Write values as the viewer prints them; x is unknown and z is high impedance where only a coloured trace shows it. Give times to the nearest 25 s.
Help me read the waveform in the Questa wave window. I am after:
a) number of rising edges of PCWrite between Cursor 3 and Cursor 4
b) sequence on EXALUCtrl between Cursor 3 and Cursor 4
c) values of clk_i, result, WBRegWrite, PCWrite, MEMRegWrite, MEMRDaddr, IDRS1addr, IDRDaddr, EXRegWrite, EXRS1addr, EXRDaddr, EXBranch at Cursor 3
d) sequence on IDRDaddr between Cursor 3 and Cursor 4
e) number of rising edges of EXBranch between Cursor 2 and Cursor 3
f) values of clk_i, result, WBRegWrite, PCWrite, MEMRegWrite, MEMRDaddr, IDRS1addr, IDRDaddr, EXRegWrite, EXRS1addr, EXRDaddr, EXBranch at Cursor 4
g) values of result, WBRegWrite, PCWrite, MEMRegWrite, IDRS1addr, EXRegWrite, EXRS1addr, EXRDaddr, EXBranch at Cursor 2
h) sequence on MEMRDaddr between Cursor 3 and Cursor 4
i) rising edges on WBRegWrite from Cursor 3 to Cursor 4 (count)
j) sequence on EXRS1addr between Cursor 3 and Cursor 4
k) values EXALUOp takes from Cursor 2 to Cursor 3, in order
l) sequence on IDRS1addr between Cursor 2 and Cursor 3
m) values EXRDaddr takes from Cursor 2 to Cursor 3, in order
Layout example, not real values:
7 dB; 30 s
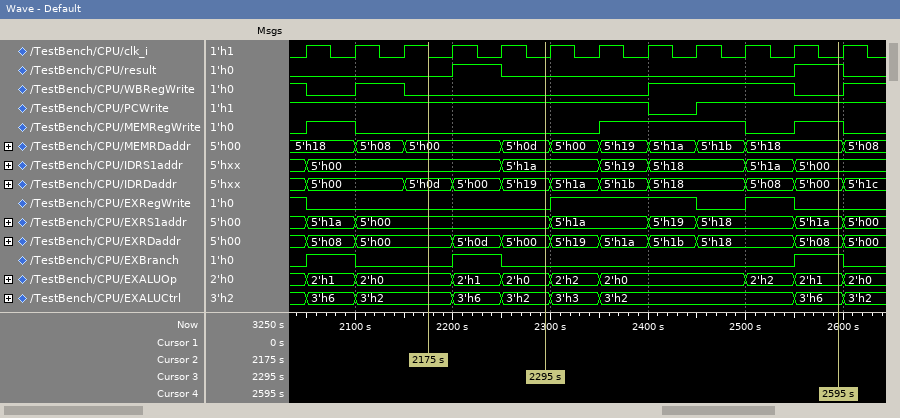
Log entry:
1; 3'h2, 3'h3, 3'h2, 3'h6; clk_i=0, result=0, WBRegWrite=0, PCWrite=1, MEMRegWrite=0, MEMRDaddr=5'h0d, IDRS1addr=5'h1a, IDRDaddr=5'h19, EXRegWrite=0, EXRS1addr=5'h00, EXRDaddr=5'h00, EXBranch=0; 5'h19, 5'h1a, 5'h1b, 5'h18, 5'h08, 5'h00; 1; clk_i=0, result=1, WBRegWrite=0, PCWrite=1, MEMRegWrite=1, MEMRDaddr=5'h18, IDRS1addr=5'h00, IDRDaddr=5'h00, EXRegWrite=0, EXRS1addr=5'h1a, EXRDaddr=5'h08, EXBranch=1; result=0, WBRegWrite=0, PCWrite=1, MEMRegWrite=0, IDRS1addr=5'h00, EXRegWrite=0, EXRS1addr=5'h00, EXRDaddr=5'h00, EXBranch=0; 5'h0d, 5'h00, 5'h19, 5'h1a, 5'h1b, 5'h18; 1; 5'h00, 5'h1a, 5'h19, 5'h18, 5'h1a; 2'h0, 2'h1, 2'h0; 5'h00, 5'h1a; 5'h00, 5'h0d, 5'h00
